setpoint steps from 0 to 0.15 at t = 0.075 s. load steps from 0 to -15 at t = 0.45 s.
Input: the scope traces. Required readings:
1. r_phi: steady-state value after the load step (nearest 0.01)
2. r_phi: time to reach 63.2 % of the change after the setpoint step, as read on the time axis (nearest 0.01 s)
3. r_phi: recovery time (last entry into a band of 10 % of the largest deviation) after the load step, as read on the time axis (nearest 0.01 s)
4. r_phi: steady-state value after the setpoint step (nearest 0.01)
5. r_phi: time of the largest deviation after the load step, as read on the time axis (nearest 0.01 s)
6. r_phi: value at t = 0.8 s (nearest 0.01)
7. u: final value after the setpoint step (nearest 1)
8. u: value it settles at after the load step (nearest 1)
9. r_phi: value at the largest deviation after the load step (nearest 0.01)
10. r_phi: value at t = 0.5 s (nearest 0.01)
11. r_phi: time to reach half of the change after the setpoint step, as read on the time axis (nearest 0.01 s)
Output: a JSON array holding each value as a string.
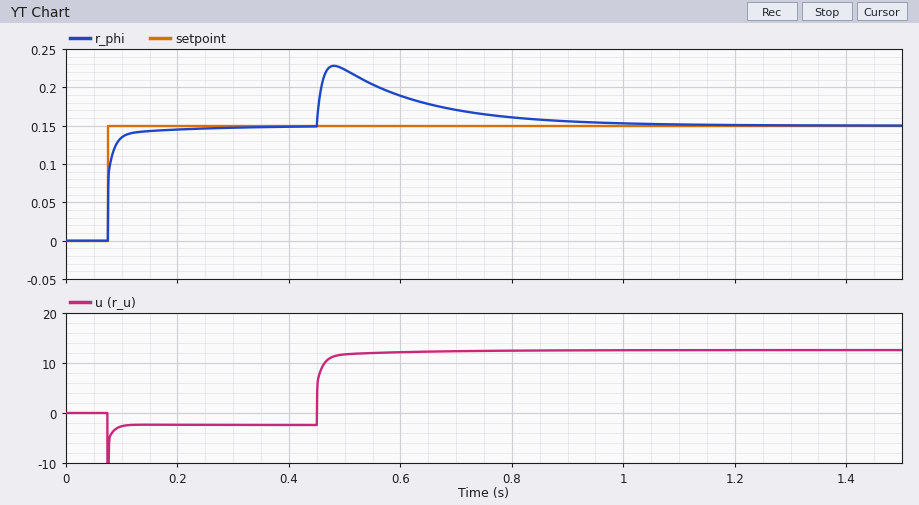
["0.15", "0.08 s", "0.85 s", "0.15", "0.48 s", "0.16", "-2", "13", "0.23", "0.22", "0.08 s"]
